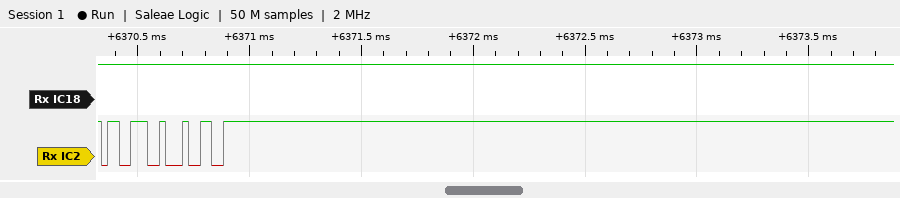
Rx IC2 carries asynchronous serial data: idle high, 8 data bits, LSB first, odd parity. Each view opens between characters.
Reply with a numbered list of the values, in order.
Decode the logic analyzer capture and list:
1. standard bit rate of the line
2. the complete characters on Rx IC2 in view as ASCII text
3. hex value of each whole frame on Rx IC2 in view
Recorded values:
1. 38400 baud
2. "sd"
3. 73, 64
